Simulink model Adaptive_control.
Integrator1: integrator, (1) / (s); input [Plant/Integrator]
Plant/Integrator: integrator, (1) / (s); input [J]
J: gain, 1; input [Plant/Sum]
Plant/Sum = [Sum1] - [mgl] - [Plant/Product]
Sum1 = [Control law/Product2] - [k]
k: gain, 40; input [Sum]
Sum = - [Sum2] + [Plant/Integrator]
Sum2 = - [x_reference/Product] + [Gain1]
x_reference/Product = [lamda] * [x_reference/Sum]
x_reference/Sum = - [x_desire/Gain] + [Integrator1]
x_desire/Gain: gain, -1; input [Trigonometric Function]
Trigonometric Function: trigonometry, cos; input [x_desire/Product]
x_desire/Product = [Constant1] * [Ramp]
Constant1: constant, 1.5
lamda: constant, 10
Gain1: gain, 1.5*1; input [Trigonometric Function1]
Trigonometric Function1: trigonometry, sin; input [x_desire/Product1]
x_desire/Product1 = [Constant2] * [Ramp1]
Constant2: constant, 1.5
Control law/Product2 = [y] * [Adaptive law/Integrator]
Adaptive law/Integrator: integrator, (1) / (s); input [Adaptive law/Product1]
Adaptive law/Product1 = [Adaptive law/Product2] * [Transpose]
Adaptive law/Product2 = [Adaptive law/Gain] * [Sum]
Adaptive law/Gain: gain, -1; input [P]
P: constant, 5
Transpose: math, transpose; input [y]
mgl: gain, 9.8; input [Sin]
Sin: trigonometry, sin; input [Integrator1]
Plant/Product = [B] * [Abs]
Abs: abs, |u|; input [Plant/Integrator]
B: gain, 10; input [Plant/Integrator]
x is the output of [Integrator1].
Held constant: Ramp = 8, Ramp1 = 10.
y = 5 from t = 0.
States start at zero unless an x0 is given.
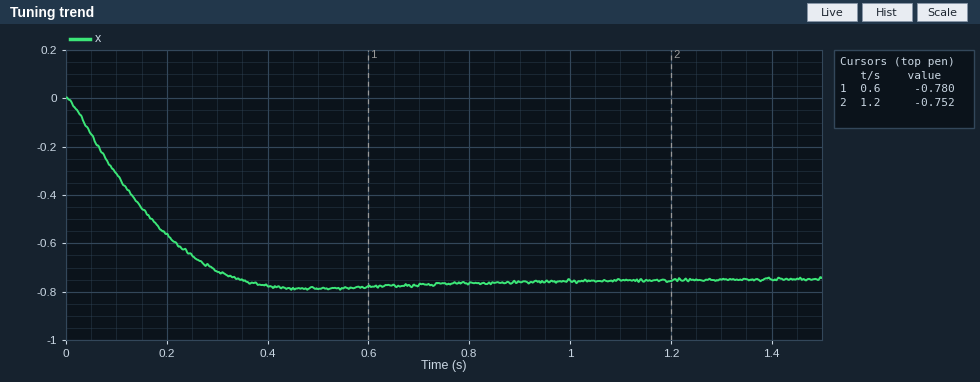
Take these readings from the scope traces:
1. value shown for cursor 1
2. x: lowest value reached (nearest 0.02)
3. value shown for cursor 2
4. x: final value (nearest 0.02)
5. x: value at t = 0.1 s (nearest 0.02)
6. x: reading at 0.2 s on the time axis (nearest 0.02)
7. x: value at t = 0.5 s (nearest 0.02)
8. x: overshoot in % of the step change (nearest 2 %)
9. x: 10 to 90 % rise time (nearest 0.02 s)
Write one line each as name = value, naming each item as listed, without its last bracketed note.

value shown for cursor 1 = -0.780
x: lowest value reached = -0.78
value shown for cursor 2 = -0.752
x: final value = -0.74
x: value at t = 0.1 s = -0.32
x: reading at 0.2 s on the time axis = -0.56
x: value at t = 0.5 s = -0.78
x: overshoot in % of the step change = 6 %
x: 10 to 90 % rise time = 0.24 s
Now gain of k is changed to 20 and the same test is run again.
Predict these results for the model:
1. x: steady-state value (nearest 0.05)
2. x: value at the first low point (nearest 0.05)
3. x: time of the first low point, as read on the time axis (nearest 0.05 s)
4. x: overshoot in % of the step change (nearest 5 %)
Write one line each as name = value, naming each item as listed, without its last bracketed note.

x: steady-state value = -0.75
x: value at the first low point = -0.85
x: time of the first low point, as read on the time axis = 0.45 s
x: overshoot in % of the step change = 15 %
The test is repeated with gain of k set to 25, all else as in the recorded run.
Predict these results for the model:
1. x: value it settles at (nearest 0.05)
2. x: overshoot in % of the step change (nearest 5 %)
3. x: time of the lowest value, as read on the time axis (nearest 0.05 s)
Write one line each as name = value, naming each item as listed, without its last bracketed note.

x: value it settles at = -0.75
x: overshoot in % of the step change = 10 %
x: time of the lowest value, as read on the time axis = 0.45 s
